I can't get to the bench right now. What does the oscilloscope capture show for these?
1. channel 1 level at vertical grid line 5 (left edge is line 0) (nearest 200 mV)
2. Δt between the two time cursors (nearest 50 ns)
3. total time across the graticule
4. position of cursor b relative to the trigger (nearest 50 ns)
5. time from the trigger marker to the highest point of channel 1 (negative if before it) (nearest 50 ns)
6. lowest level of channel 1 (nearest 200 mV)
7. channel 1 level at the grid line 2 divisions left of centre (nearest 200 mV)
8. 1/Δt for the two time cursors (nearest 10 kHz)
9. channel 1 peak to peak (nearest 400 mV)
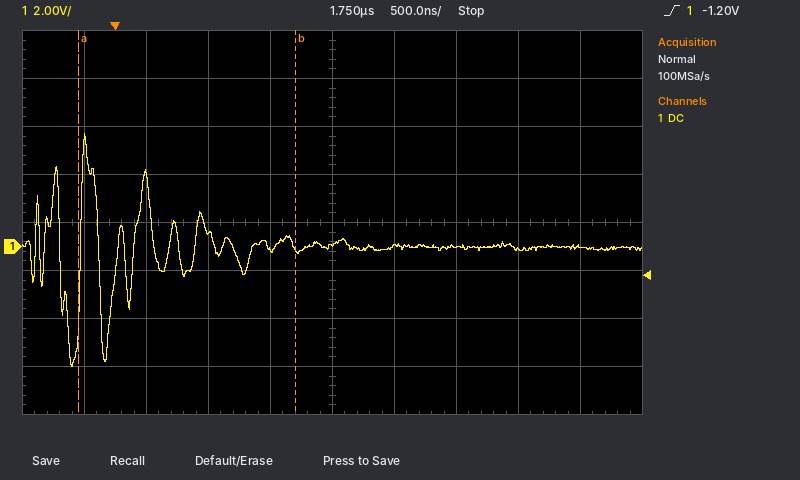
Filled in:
0.0 V
1.75 µs
5 µs
+1.45 µs
-250 ns
-5.0 V
600 mV
570 kHz
9.6 V
